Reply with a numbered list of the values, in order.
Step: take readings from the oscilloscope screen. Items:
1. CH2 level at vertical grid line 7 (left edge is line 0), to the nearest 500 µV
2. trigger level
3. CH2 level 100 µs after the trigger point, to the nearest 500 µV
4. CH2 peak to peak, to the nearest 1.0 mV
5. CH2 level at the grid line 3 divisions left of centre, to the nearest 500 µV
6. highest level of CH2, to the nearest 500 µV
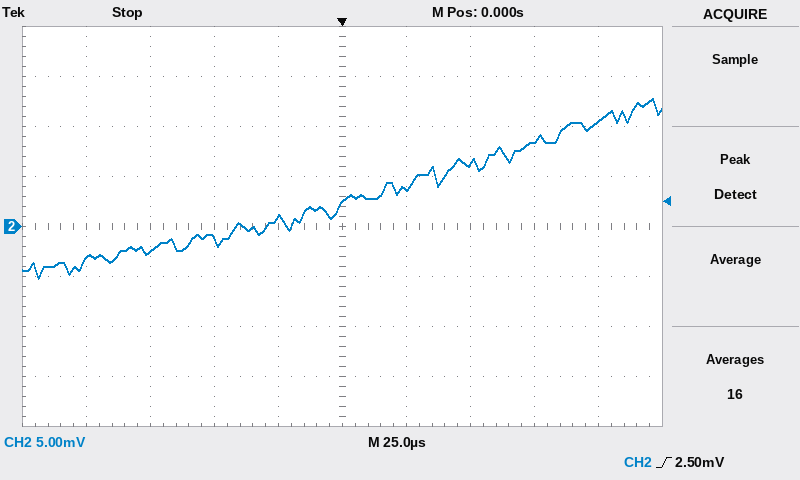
1. 6.5 mV
2. 2.50 mV
3. 10.5 mV
4. 18.0 mV
5. -2.5 mV
6. 13.0 mV
